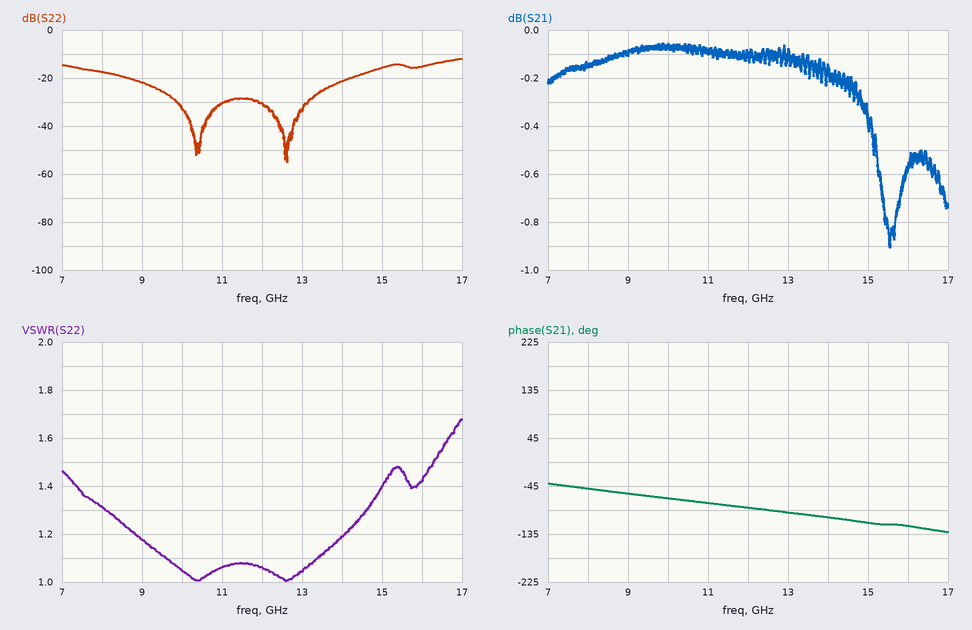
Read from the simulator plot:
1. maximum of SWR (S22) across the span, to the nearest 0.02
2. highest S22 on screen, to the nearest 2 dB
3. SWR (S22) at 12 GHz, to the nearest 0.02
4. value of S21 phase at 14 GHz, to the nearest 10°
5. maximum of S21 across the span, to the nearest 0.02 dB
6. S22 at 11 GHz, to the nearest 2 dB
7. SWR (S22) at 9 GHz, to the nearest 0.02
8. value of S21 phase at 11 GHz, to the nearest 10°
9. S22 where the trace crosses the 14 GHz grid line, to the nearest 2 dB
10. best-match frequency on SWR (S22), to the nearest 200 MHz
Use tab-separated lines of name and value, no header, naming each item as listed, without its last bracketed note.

maximum of SWR (S22) across the span, to the nearest 0.02	1.68
highest S22 on screen, to the nearest 2 dB	-12 dB
SWR (S22) at 12 GHz, to the nearest 0.02	1.06
value of S21 phase at 14 GHz, to the nearest 10°	-100°
maximum of S21 across the span, to the nearest 0.02 dB	-0.06 dB
S22 at 11 GHz, to the nearest 2 dB	-30 dB
SWR (S22) at 9 GHz, to the nearest 0.02	1.18
value of S21 phase at 11 GHz, to the nearest 10°	-80°
S22 where the trace crosses the 14 GHz grid line, to the nearest 2 dB	-22 dB
best-match frequency on SWR (S22), to the nearest 200 MHz	12.6 GHz
